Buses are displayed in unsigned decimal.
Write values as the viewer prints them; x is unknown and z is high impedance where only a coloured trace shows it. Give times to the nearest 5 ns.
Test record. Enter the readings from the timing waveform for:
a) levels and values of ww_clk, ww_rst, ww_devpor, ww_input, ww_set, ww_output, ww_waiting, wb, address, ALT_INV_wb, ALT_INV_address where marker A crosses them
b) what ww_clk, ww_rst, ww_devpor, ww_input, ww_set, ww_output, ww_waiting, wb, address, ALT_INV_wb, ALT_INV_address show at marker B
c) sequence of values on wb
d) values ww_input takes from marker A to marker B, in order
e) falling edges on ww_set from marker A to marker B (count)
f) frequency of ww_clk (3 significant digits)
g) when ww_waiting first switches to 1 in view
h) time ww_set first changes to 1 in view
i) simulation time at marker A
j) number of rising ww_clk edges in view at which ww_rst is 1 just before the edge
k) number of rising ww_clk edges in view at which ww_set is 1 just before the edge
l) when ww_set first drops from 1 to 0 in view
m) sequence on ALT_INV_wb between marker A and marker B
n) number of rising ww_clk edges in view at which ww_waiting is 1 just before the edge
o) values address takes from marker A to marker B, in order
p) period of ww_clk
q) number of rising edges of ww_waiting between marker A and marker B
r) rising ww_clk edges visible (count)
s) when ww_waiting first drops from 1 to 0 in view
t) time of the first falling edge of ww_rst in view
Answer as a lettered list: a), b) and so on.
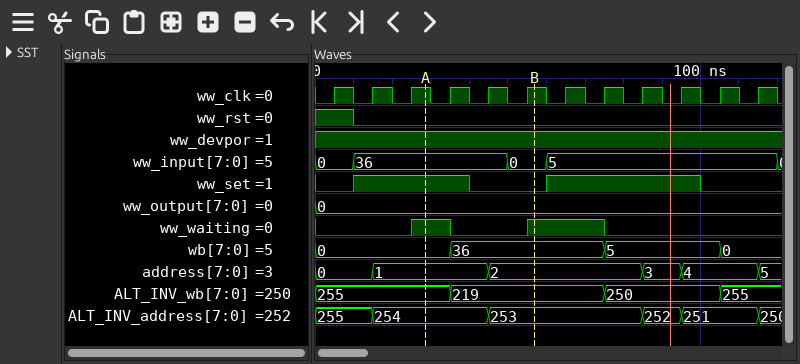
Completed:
a) ww_clk=1, ww_rst=0, ww_devpor=1, ww_input=36, ww_set=1, ww_output=0, ww_waiting=1, wb=0, address=1, ALT_INV_wb=255, ALT_INV_address=254
b) ww_clk=1, ww_rst=0, ww_devpor=1, ww_input=0, ww_set=0, ww_output=0, ww_waiting=1, wb=36, address=2, ALT_INV_wb=219, ALT_INV_address=253
c) 0, 36, 5, 0
d) 36, 0
e) 1
f) 100 MHz
g) 25 ns
h) 10 ns
i) 30 ns
j) 1
k) 7
l) 40 ns
m) 255, 219
n) 3
o) 1, 2
p) 10 ns
q) 1
r) 12
s) 35 ns
t) 10 ns
